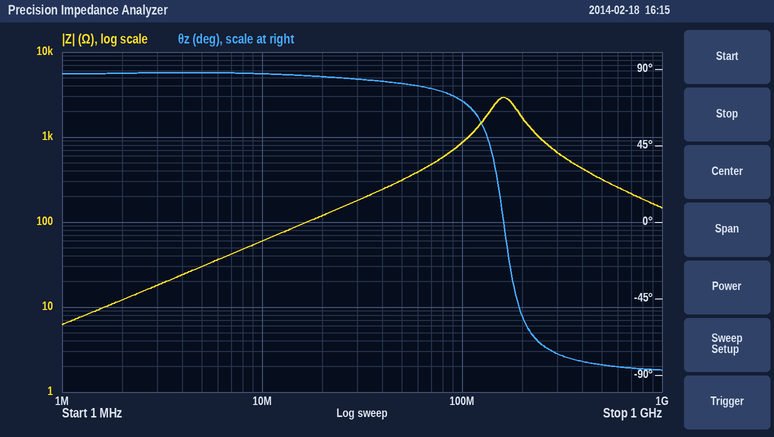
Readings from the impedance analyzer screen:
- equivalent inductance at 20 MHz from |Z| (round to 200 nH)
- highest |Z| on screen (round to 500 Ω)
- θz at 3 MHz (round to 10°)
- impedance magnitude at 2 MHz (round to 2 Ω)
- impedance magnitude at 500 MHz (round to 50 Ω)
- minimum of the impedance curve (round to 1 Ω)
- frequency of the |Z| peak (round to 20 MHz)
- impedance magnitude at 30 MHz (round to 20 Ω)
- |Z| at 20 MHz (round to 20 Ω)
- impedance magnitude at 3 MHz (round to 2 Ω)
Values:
1.0 µH
3.0 kΩ
90°
12 Ω
300 Ω
6 Ω
160 MHz
180 Ω
120 Ω
18 Ω
